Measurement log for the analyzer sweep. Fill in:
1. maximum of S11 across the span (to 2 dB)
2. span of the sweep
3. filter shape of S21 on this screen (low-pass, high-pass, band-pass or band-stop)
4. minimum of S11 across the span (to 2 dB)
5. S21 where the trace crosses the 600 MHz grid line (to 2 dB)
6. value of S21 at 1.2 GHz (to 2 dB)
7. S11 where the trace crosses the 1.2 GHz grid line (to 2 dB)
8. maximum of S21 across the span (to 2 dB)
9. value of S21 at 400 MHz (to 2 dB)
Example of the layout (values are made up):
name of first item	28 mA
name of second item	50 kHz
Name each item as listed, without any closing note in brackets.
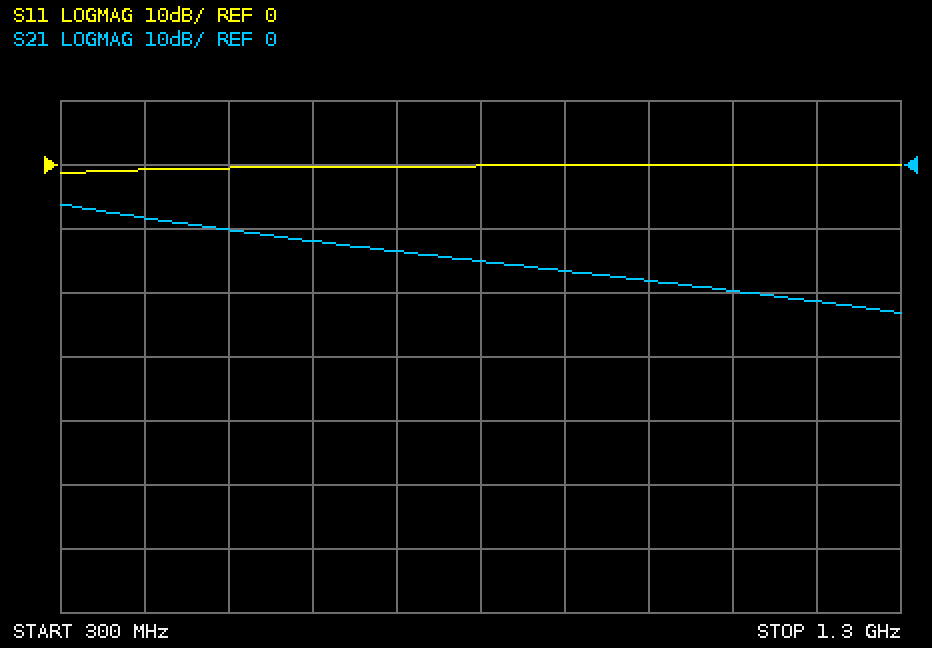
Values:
maximum of S11 across the span	0 dB
span of the sweep	1 GHz
filter shape of S21 on this screen	low-pass
minimum of S11 across the span	-2 dB
S21 where the trace crosses the 600 MHz grid line	-12 dB
value of S21 at 1.2 GHz	-22 dB
S11 where the trace crosses the 1.2 GHz grid line	0 dB
maximum of S21 across the span	-6 dB
value of S21 at 400 MHz	-8 dB
